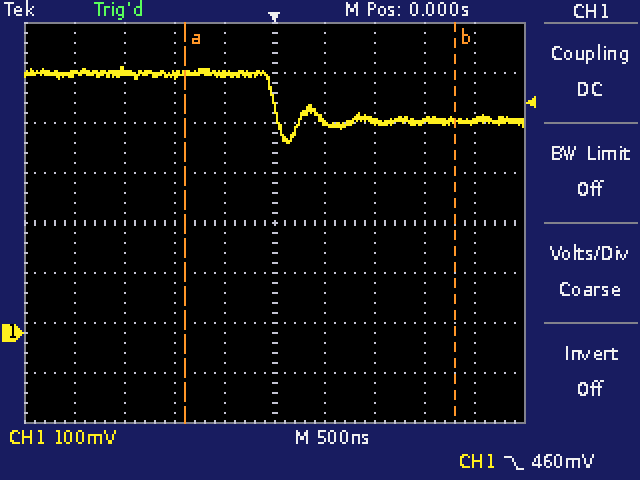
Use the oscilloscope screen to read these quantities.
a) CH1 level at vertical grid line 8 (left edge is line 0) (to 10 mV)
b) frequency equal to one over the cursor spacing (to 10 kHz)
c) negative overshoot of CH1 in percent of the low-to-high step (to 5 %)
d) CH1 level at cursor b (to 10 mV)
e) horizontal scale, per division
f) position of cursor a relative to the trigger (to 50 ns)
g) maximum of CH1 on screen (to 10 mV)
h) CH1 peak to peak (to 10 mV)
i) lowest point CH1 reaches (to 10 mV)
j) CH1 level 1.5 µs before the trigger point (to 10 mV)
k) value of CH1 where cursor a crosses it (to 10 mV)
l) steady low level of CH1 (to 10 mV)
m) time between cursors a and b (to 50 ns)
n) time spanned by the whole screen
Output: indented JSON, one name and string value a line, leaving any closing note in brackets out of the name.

{
  "CH1 level at vertical grid line 8 (left edge is line 0)": "420 mV",
  "frequency equal to one over the cursor spacing": "370 kHz",
  "negative overshoot of CH1 in percent of the low-to-high step": "45 %",
  "CH1 level at cursor b": "420 mV",
  "horizontal scale, per division": "500 ns",
  "position of cursor a relative to the trigger": "-900 ns",
  "maximum of CH1 on screen": "530 mV",
  "CH1 peak to peak": "150 mV",
  "lowest point CH1 reaches": "380 mV",
  "CH1 level 1.5 µs before the trigger point": "520 mV",
  "value of CH1 where cursor a crosses it": "520 mV",
  "steady low level of CH1": "420 mV",
  "time between cursors a and b": "2.70 µs",
  "time spanned by the whole screen": "5 µs"
}
